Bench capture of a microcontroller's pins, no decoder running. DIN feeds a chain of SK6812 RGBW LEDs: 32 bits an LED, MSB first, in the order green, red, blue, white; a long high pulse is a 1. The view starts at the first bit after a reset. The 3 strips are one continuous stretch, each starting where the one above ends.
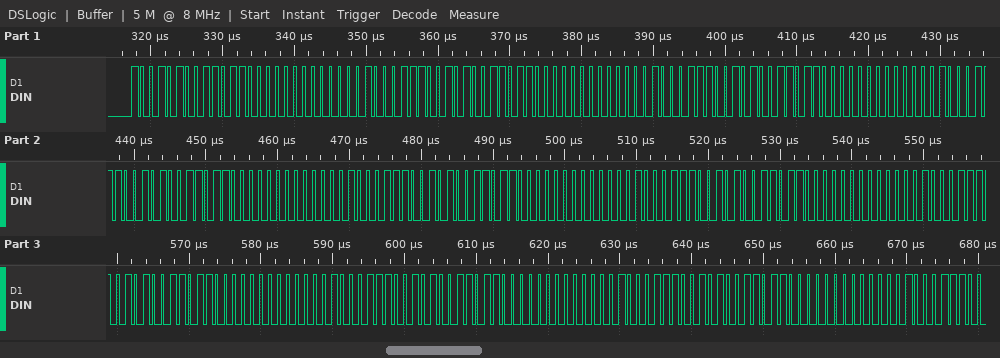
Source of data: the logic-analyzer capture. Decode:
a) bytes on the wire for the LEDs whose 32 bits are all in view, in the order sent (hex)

94 D8 00 23 94 D8 00 23 94 D8 00 23 94 D8 00 23 94 D8 00 23 94 D8 00 23 94 D8 00 23 94 D8 00 23 94 D8 00 23
